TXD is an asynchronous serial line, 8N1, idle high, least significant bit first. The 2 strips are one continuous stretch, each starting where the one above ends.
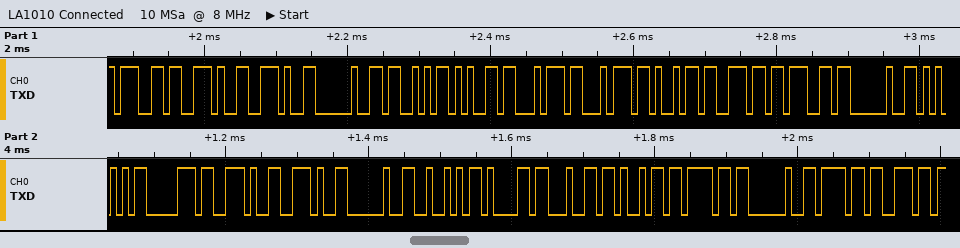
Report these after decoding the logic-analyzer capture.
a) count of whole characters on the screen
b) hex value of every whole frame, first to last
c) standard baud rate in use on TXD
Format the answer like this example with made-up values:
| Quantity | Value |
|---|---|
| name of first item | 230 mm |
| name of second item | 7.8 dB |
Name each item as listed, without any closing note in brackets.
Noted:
| Quantity | Value |
|---|---|
| count of whole characters on the screen | 25 |
| hex value of every whole frame, first to last | 67 2E 2E 20 53 65 74 74 69 6E 67 20 55 70 2E 2E 20 52 61 64 69 6F 20 6F 6E |
| standard baud rate in use on TXD | 115200 baud |
